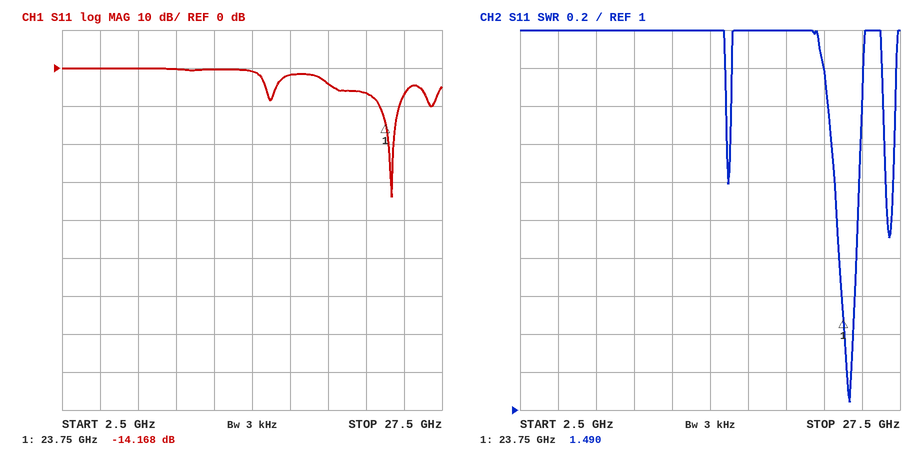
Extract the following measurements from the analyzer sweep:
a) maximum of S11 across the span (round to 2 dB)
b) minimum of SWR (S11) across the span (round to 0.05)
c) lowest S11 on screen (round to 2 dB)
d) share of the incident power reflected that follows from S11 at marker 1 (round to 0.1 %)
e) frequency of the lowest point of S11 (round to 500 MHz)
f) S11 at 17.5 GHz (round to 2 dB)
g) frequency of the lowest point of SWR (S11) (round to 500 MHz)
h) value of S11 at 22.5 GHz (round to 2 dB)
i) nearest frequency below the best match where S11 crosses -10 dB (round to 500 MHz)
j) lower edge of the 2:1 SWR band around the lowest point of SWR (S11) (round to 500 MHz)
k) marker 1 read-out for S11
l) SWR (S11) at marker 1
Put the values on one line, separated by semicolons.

0 dB; 1.05; -34 dB; 3.8 %; 24.0 GHz; -2 dB; 24.0 GHz; -6 dB; 23.5 GHz; 23.5 GHz; -14.168 dB; 1.490
